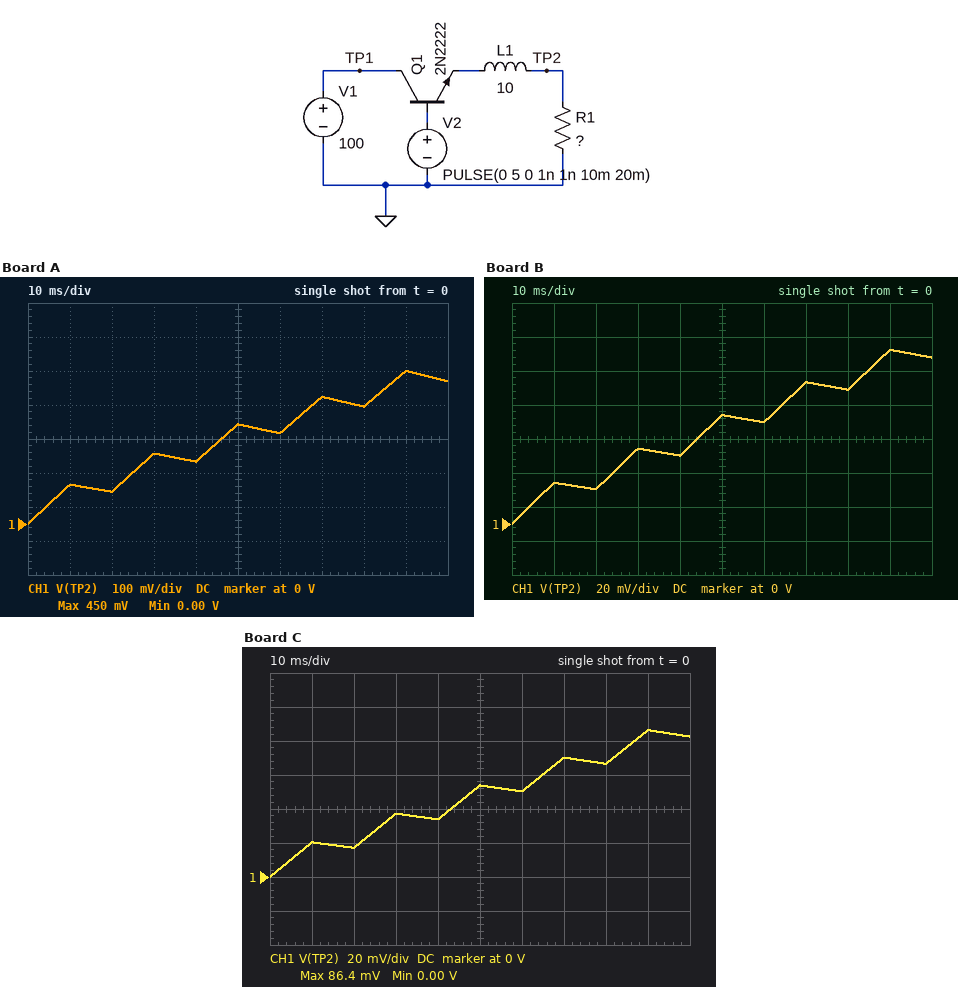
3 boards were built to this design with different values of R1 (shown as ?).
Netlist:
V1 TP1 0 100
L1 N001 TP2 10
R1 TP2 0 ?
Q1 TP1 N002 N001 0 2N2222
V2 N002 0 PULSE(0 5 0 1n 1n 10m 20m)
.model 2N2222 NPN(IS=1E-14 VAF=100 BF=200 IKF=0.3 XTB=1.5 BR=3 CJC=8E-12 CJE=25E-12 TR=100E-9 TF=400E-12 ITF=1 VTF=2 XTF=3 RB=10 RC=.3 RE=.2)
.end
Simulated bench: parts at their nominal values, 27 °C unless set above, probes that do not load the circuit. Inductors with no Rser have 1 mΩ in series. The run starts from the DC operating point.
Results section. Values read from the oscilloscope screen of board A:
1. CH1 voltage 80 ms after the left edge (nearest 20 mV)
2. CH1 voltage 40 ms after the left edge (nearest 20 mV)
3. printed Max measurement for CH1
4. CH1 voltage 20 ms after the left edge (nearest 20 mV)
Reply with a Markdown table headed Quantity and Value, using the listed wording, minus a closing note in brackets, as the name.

| Quantity | Value |
|---|---|
| CH1 voltage 80 ms after the left edge | 340 mV |
| CH1 voltage 40 ms after the left edge | 180 mV |
| printed Max measurement for CH1 | 450 mV |
| CH1 voltage 20 ms after the left edge | 100 mV |
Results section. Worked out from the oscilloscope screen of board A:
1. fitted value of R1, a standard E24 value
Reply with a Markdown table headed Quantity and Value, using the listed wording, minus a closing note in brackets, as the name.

| Quantity | Value |
|---|---|
| fitted value of R1, a standard E24 value | 27 Ω |
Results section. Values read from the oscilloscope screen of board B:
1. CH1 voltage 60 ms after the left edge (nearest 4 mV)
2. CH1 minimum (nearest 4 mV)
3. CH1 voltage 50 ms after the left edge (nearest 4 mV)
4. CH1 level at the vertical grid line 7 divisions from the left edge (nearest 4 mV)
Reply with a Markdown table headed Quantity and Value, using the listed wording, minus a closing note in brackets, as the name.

| Quantity | Value |
|---|---|
| CH1 voltage 60 ms after the left edge | 60 mV |
| CH1 minimum | 0 V |
| CH1 voltage 50 ms after the left edge | 64 mV |
| CH1 level at the vertical grid line 7 divisions from the left edge | 84 mV |
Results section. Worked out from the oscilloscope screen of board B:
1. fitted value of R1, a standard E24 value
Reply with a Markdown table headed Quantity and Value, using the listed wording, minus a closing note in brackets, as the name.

| Quantity | Value |
|---|---|
| fitted value of R1, a standard E24 value | 5.6 Ω |
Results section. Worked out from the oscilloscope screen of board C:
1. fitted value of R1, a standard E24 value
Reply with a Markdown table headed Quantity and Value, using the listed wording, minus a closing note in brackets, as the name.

| Quantity | Value |
|---|---|
| fitted value of R1, a standard E24 value | 4.7 Ω |
